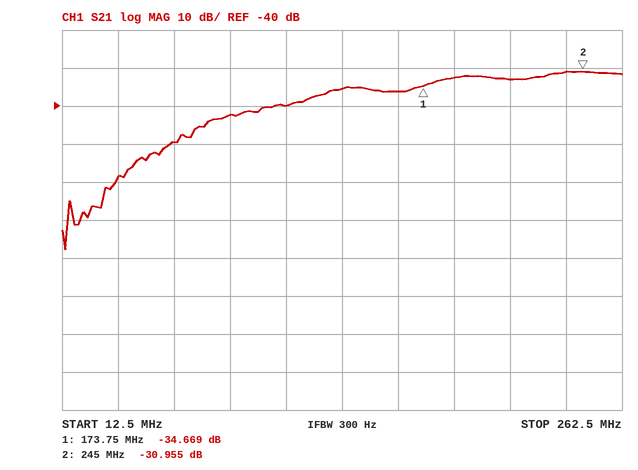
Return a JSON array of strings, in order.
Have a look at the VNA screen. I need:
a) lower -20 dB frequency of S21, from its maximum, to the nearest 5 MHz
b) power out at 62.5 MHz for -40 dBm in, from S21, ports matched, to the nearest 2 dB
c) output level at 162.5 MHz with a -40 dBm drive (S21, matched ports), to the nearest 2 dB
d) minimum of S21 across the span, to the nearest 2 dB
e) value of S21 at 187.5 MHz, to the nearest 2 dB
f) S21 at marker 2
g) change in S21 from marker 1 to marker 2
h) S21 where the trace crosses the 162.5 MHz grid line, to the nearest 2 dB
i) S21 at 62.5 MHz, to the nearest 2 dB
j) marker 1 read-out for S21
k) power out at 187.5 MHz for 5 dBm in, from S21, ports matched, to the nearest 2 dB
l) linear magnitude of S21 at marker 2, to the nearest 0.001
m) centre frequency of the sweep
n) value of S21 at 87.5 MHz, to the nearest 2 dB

["60 MHz", "-90 dBm", "-76 dBm", "-78 dB", "-32 dB", "-30.955 dB", "3.714 dB", "-36 dB", "-50 dB", "-34.669 dB", "-28 dBm", "0.028", "137.5 MHz", "-42 dB"]
